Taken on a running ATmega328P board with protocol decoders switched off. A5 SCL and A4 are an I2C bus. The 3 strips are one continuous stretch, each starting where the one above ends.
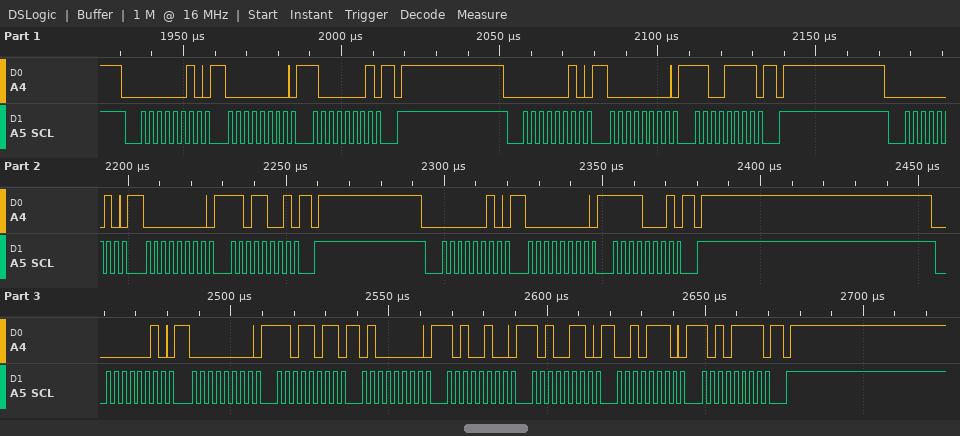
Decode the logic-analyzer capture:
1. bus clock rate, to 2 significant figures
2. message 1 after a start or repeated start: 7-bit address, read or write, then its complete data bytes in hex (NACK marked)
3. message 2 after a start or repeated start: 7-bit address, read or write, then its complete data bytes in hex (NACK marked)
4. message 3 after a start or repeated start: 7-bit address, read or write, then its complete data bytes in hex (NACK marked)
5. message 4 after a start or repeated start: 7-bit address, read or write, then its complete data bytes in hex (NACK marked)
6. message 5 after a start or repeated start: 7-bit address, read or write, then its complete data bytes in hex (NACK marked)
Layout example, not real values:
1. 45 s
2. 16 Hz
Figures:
1. 400 kHz
2. 0x01 write: 00 81
3. 0x01 write: 00 CF
4. 0x01 write: 00 D9
5. 0x01 write: 00 F1
6. 0x01 write: 00 DB 40 A4 A6 2E AF
